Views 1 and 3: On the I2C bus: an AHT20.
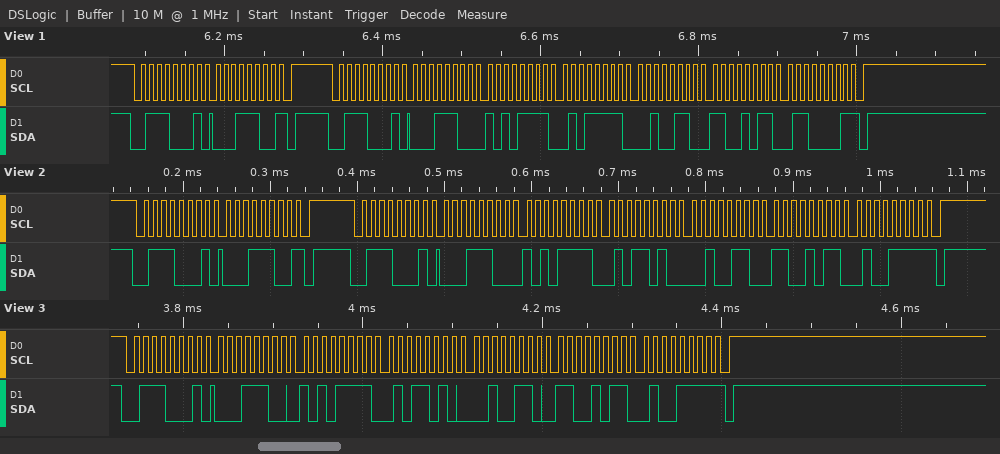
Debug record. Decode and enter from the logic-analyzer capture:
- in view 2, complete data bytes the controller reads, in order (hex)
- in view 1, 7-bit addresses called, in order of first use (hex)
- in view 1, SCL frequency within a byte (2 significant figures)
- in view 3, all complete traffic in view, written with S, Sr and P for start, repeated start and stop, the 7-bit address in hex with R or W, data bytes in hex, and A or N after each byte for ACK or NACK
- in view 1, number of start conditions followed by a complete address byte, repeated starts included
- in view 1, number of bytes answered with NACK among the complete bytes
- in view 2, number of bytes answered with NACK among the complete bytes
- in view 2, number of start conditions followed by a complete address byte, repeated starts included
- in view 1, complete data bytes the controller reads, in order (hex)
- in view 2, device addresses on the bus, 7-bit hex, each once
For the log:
1C 1C AF 5A 26 CB 4F
0x38
100 kHz
S 38R A 1C A AF A 5A A 26 A CB A 4F N P
2
2
2
2
1C 1C AF 5F 26 CB 61
0x38
